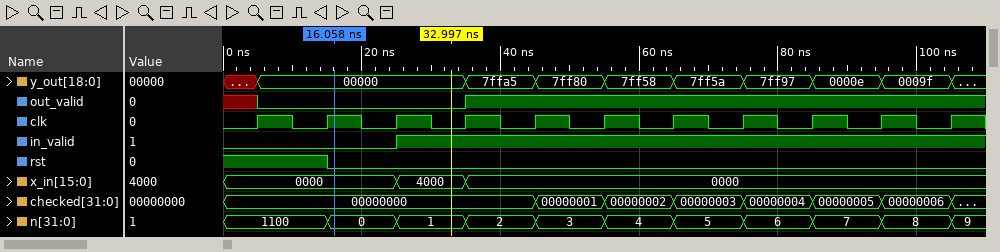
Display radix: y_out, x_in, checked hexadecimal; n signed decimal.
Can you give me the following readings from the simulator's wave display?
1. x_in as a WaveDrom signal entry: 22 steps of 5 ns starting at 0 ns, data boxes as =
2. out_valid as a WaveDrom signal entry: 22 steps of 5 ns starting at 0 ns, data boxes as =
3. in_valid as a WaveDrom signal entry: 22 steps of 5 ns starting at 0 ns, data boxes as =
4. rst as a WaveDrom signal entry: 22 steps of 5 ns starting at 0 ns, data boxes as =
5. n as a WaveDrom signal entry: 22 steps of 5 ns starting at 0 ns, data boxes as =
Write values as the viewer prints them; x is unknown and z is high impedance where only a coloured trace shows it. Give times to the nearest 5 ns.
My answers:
{name: 'x_in', wave: '=....=.=..............', data: '0000 4000 0000'}
{name: 'out_valid', wave: 'x0.....1..............'}
{name: 'in_valid', wave: '0....1................'}
{name: 'rst', wave: '1..0..................'}
{name: 'n', wave: '=..=.=.=.=.=.=.=.=.=.=', data: '1100 0 1 2 3 4 5 6 7 8 9'}
